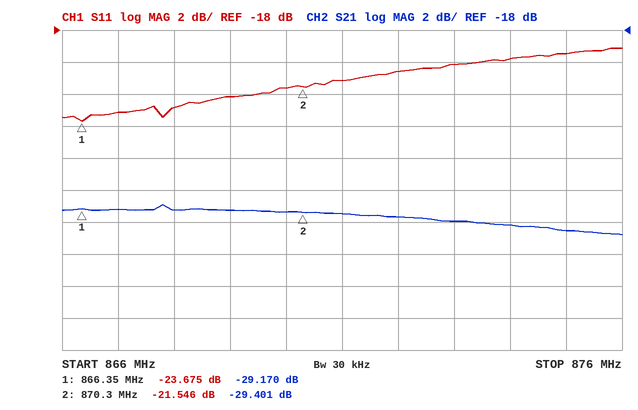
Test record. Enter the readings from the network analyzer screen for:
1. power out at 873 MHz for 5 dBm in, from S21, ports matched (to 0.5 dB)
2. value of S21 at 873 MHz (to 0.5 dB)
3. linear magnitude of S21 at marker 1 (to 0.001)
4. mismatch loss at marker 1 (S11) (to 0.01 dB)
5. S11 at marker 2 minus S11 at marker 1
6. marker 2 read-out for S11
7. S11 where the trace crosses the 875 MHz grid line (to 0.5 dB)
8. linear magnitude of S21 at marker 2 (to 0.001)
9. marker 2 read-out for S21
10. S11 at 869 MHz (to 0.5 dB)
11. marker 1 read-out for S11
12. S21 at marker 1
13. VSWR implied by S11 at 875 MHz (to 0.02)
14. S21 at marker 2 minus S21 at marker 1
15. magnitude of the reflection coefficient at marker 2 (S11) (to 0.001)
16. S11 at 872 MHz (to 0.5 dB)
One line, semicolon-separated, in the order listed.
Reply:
-25.0 dBm; -30.0 dB; 0.035; 0.02 dB; 2.129 dB; -21.546 dB; -19.5 dB; 0.034; -29.401 dB; -22.0 dB; -23.675 dB; -29.170 dB; 1.24; -0.231 dB; 0.084; -20.5 dB
